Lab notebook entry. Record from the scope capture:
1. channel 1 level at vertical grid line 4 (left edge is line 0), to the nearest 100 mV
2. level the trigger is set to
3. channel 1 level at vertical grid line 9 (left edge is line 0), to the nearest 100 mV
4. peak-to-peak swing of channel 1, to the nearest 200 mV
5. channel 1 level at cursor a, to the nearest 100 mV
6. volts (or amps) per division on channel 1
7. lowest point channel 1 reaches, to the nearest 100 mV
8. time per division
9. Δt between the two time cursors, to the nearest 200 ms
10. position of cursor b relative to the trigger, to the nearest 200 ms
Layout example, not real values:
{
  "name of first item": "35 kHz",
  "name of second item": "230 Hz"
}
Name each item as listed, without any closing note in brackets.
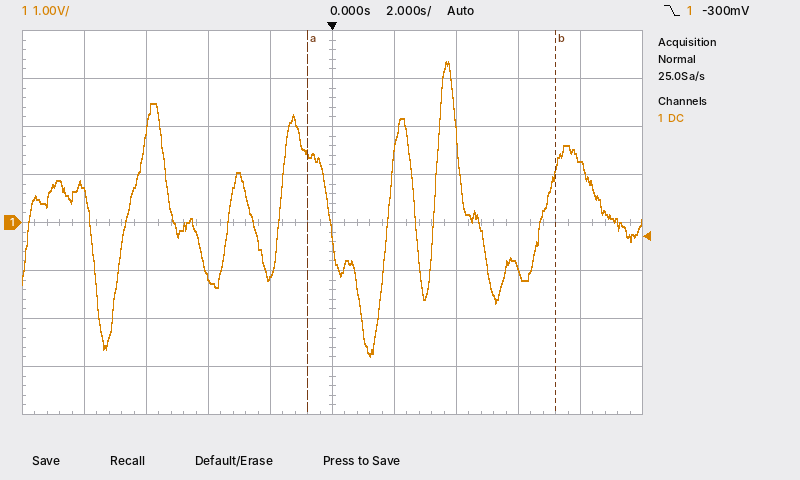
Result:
{
  "channel 1 level at vertical grid line 4 (left edge is line 0), to the nearest 100 mV": "-1.1 V",
  "level the trigger is set to": "-300 mV",
  "channel 1 level at vertical grid line 9 (left edge is line 0), to the nearest 100 mV": "1.3 V",
  "peak-to-peak swing of channel 1, to the nearest 200 mV": "6.2 V",
  "channel 1 level at cursor a, to the nearest 100 mV": "1.4 V",
  "volts (or amps) per division on channel 1": "1 V",
  "lowest point channel 1 reaches, to the nearest 100 mV": "-2.8 V",
  "time per division": "2 s",
  "Δt between the two time cursors, to the nearest 200 ms": "8.0 s",
  "position of cursor b relative to the trigger, to the nearest 200 ms": "+7.2 s"
}
